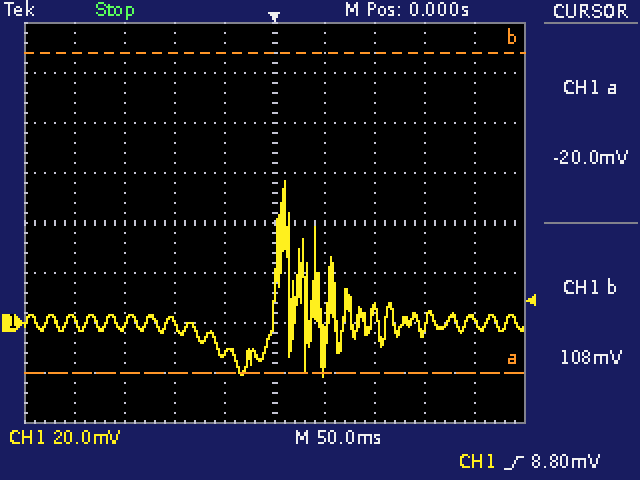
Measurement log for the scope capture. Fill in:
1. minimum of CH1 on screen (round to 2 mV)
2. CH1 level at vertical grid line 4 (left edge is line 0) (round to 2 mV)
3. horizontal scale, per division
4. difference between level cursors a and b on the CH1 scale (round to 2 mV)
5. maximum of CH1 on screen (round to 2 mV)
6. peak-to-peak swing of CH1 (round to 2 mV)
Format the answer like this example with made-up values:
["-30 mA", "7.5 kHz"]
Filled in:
["-22 mV", "-12 mV", "50 ms", "128 mV", "56 mV", "78 mV"]
